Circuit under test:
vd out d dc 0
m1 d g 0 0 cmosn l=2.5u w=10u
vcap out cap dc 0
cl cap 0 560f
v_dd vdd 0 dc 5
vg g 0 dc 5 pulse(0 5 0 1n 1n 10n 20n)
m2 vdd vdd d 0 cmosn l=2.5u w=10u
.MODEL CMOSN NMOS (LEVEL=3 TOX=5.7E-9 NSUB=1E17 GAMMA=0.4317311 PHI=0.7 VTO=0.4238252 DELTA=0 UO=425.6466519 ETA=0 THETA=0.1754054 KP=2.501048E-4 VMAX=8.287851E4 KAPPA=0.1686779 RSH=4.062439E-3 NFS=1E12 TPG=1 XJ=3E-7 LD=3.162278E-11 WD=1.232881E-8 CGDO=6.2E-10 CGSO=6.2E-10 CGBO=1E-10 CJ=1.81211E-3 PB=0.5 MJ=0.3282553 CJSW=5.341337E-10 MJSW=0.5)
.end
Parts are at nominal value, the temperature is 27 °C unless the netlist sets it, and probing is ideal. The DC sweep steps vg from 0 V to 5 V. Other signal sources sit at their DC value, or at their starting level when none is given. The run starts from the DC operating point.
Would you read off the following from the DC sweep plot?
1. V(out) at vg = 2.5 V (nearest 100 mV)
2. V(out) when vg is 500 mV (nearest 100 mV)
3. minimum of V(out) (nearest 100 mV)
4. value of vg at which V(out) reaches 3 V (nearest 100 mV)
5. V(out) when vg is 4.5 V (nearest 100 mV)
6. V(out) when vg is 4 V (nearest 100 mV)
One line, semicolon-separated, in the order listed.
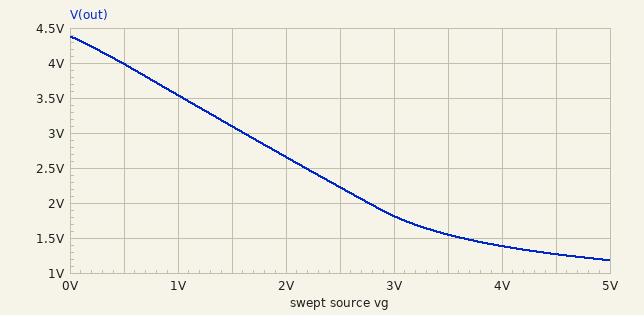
2.2 V; 4.0 V; 1.2 V; 1.6 V; 1.3 V; 1.4 V
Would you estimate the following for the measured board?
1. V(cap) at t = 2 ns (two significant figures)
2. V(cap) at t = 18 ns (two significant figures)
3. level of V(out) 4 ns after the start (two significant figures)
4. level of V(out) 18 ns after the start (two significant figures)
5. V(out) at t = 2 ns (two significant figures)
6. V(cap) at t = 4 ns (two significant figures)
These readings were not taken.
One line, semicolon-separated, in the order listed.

1.2 V; 3.9 V; 1.2 V; 3.9 V; 1.2 V; 1.2 V
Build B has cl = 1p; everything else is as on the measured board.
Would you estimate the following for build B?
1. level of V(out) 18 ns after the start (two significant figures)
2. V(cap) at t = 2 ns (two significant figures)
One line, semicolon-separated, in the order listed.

3.7 V; 1.5 V
